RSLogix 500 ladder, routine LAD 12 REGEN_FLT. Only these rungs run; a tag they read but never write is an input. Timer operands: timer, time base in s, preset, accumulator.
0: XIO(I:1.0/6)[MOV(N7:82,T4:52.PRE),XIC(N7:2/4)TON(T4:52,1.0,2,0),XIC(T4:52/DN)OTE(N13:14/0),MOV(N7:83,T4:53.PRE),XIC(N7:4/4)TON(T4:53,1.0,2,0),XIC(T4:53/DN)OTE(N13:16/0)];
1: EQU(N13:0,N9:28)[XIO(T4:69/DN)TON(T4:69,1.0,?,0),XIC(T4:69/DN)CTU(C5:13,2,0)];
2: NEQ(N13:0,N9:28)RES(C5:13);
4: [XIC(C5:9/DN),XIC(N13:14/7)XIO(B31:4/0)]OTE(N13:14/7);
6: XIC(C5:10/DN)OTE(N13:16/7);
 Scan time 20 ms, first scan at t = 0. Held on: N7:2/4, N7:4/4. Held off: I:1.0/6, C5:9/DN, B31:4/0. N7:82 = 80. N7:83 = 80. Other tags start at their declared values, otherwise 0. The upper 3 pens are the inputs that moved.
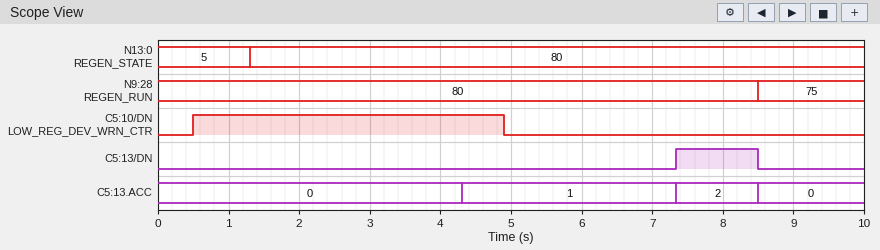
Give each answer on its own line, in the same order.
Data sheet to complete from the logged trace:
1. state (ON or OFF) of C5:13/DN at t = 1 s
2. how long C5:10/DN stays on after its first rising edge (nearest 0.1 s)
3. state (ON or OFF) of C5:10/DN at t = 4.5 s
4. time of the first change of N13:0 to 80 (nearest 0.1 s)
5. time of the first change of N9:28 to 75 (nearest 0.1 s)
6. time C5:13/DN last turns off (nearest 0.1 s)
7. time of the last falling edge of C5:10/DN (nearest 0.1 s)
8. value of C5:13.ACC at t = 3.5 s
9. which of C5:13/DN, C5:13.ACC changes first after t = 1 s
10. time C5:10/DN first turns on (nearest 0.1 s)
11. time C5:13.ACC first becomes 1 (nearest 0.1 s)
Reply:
OFF
4.4 s
ON
1.3 s
8.5 s
8.5 s
4.9 s
0
C5:13.ACC
0.5 s
4.3 s
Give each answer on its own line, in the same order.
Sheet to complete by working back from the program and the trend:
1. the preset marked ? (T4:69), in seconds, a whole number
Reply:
3 s
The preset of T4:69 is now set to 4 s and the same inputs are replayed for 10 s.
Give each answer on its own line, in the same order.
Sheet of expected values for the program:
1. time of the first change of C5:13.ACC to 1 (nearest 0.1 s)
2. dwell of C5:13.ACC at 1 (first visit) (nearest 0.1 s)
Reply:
5.3 s
3.2 s
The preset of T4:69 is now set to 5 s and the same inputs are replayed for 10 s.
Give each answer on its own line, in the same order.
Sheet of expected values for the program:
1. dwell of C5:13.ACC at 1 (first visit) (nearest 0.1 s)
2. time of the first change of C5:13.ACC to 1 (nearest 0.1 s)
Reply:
2.2 s
6.3 s
